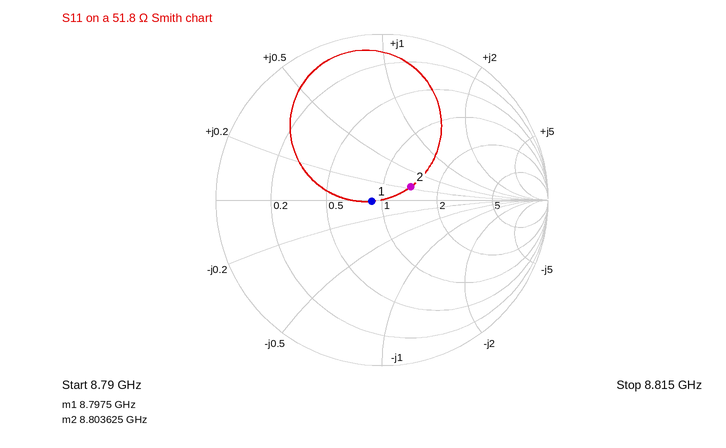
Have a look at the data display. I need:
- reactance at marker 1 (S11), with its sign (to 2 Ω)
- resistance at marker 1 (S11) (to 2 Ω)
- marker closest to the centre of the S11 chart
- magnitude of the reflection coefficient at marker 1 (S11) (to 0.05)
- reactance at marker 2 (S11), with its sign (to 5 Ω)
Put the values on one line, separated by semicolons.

0 Ω; 46 Ω; marker 1; 0.05; +10 Ω
